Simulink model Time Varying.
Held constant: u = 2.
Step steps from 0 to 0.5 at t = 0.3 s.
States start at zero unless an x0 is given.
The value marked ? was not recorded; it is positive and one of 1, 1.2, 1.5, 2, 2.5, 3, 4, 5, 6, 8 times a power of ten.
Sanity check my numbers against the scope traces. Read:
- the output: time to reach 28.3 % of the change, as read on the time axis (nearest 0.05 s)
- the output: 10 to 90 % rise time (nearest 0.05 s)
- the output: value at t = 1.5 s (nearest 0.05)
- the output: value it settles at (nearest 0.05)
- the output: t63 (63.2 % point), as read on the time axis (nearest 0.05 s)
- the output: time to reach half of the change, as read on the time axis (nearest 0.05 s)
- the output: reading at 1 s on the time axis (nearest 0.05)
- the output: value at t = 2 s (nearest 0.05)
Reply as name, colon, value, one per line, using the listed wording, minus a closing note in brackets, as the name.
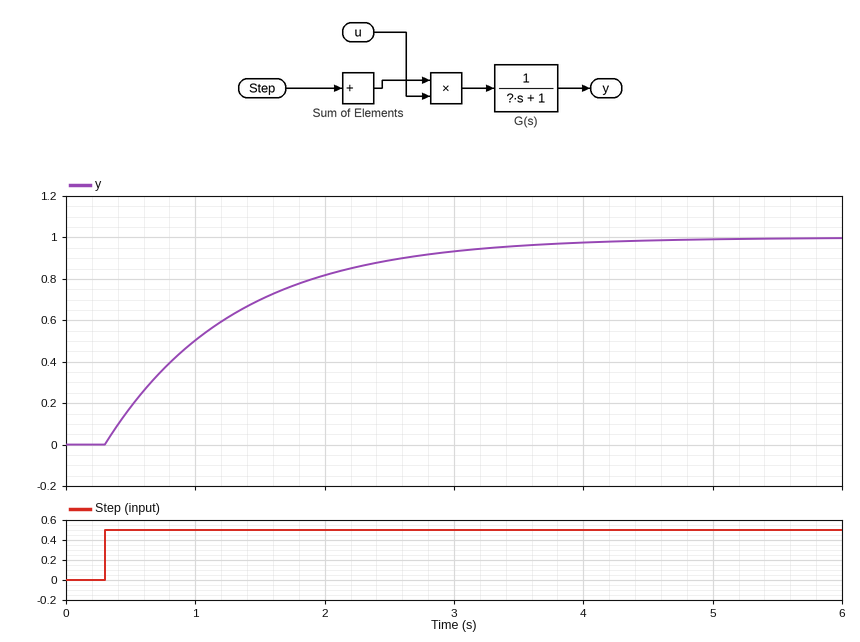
the output: time to reach 28.3 % of the change, as read on the time axis: 0.65 s
the output: 10 to 90 % rise time: 2.20 s
the output: value at t = 1.5 s: 0.70
the output: value it settles at: 1.00
the output: t63 (63.2 % point), as read on the time axis: 1.30 s
the output: time to reach half of the change, as read on the time axis: 1.00 s
the output: reading at 1 s on the time axis: 0.50
the output: value at t = 2 s: 0.80
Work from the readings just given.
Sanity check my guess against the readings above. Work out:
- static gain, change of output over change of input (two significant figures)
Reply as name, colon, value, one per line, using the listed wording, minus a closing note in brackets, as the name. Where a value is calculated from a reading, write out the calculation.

static gain, change of output over change of input: (1 - 0) / (0.5 - 0) = 2.0
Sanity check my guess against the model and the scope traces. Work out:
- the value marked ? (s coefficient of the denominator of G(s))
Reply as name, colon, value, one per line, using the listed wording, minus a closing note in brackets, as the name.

the value marked ? (s coefficient of the denominator of G(s)): 1
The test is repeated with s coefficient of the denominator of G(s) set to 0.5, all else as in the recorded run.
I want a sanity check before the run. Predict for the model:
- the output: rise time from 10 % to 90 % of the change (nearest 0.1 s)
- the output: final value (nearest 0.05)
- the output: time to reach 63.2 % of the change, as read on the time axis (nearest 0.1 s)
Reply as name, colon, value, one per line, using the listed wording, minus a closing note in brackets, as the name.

the output: rise time from 10 % to 90 % of the change: 1.1 s
the output: final value: 1.00
the output: time to reach 63.2 % of the change, as read on the time axis: 0.8 s
